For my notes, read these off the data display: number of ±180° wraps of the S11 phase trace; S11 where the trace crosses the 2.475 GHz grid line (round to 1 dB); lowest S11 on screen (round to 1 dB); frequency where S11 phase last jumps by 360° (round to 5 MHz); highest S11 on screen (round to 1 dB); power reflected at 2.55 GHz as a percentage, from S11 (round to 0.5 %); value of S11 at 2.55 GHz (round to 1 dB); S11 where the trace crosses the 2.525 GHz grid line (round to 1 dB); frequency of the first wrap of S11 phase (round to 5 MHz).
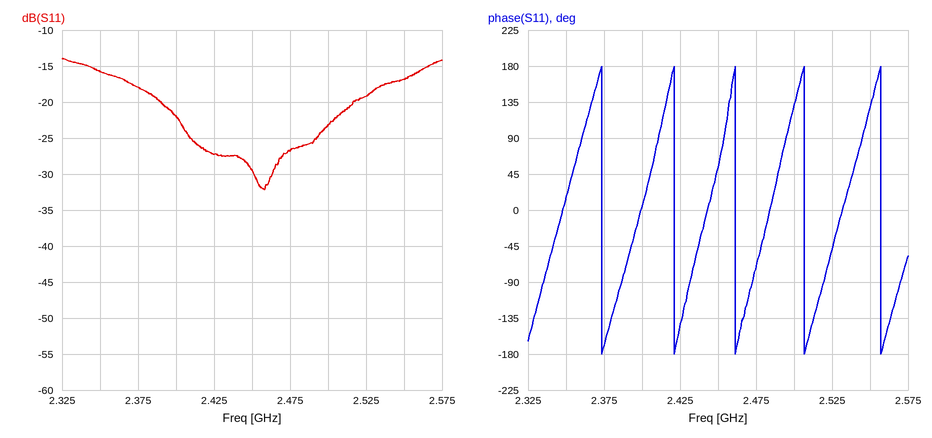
5
-27 dB
-32 dB
2.555 GHz
-14 dB
2.0 %
-17 dB
-19 dB
2.375 GHz
